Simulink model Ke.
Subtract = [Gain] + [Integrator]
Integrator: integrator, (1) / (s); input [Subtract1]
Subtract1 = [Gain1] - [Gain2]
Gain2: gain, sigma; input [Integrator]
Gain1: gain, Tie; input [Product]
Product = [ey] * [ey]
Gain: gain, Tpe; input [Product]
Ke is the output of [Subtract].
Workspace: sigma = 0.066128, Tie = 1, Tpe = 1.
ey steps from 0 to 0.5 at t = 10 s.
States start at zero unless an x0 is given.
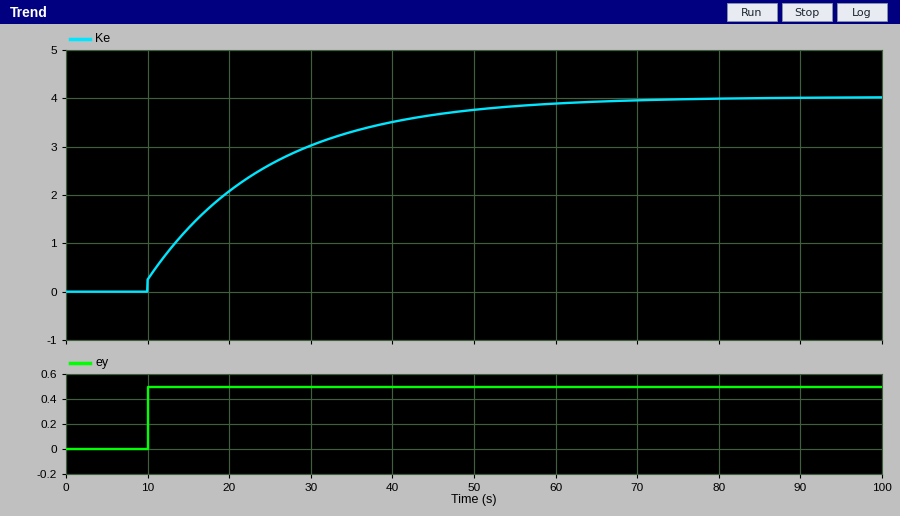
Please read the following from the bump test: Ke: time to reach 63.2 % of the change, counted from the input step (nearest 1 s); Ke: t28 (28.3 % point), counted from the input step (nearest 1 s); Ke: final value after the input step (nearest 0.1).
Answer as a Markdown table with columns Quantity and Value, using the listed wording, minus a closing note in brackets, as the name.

| Quantity | Value |
|---|---|
| Ke: time to reach 63.2 % of the change, counted from the input step | 14 s |
| Ke: t28 (28.3 % point), counted from the input step | 4 s |
| Ke: final value after the input step | 4.0 |
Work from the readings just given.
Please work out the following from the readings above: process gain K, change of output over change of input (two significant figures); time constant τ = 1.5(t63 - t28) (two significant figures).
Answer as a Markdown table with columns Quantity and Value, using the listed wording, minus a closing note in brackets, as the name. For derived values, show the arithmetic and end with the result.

| Quantity | Value |
|---|---|
| process gain K, change of output over change of input | (4 - 0) / 0.5 = 8.0 |
| time constant τ = 1.5(t63 - t28) | 1.5 × (14 - 4) = 15 s |
